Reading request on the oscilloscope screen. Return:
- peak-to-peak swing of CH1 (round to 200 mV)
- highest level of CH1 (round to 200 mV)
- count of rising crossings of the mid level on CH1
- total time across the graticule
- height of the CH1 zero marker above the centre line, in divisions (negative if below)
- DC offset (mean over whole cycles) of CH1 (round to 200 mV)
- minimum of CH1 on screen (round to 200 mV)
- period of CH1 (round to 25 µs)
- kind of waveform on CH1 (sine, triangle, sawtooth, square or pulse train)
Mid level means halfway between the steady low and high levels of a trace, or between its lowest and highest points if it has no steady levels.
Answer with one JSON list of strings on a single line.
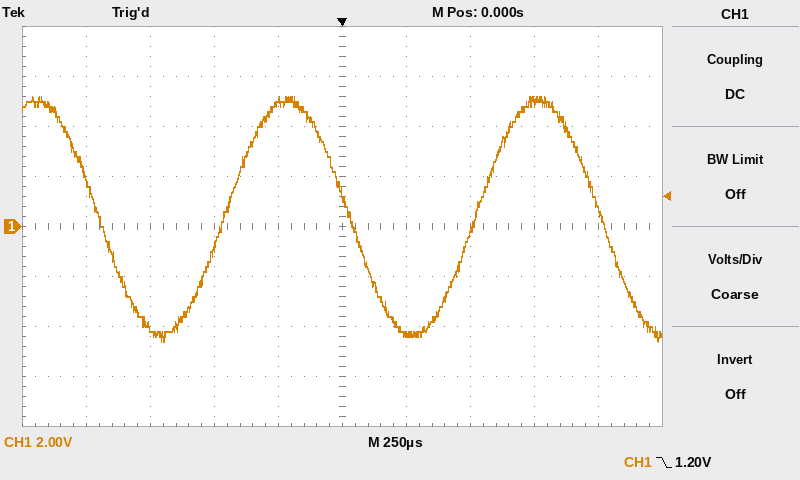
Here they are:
["9.8 V", "5.2 V", "2", "2.5 ms", "0.0 div", "400 mV", "-4.6 V", "975 µs", "sine"]
